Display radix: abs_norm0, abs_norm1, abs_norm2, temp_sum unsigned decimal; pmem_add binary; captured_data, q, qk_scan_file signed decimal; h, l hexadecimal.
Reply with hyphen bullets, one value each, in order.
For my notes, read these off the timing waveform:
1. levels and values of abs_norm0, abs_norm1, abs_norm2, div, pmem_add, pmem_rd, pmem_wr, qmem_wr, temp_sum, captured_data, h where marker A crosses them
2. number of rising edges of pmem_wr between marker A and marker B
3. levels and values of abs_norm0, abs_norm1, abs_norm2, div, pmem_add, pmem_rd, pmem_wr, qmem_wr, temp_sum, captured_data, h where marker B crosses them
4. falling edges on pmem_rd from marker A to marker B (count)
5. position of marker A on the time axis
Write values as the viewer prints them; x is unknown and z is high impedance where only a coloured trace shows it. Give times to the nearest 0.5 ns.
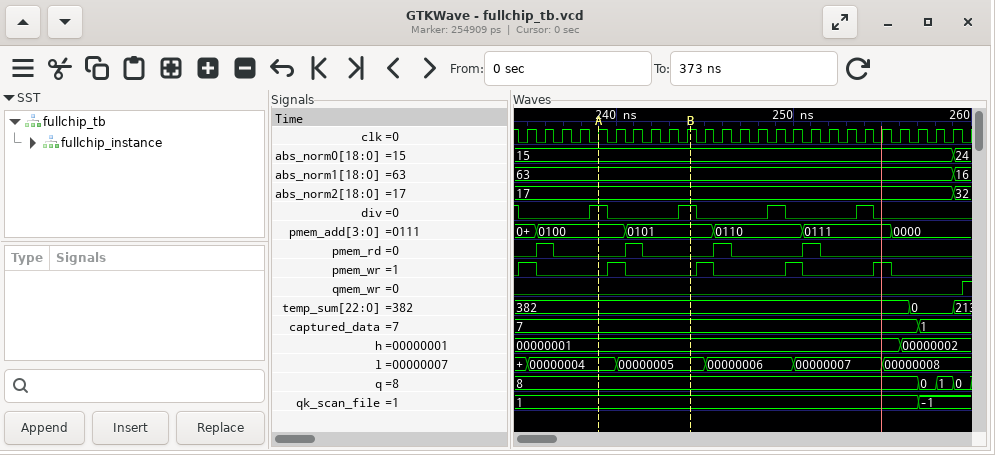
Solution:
- abs_norm0=15, abs_norm1=63, abs_norm2=17, div=1, pmem_add=0100, pmem_rd=0, pmem_wr=0, qmem_wr=0, temp_sum=382, captured_data=7, h=00000001
- 1
- abs_norm0=15, abs_norm1=63, abs_norm2=17, div=1, pmem_add=0101, pmem_rd=0, pmem_wr=0, qmem_wr=0, temp_sum=382, captured_data=7, h=00000001
- 1
- 239 ns
